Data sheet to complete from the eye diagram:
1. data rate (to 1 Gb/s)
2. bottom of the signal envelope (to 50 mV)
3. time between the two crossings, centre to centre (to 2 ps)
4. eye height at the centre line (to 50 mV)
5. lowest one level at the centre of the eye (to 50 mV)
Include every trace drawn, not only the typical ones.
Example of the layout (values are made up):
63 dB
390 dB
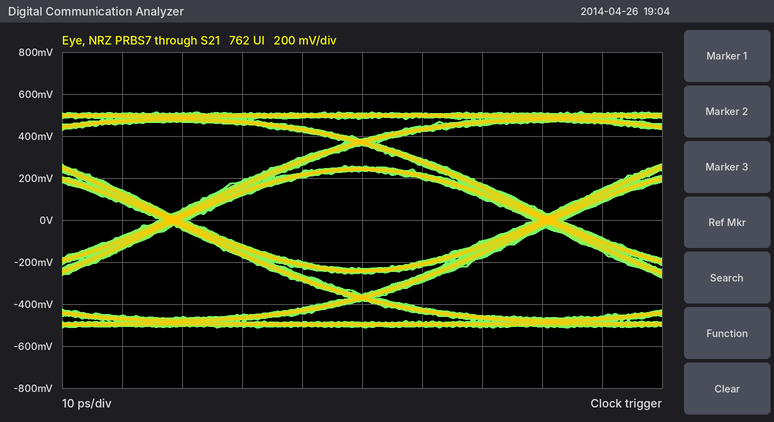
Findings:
16 Gb/s
-500 mV
62 ps
450 mV
250 mV
